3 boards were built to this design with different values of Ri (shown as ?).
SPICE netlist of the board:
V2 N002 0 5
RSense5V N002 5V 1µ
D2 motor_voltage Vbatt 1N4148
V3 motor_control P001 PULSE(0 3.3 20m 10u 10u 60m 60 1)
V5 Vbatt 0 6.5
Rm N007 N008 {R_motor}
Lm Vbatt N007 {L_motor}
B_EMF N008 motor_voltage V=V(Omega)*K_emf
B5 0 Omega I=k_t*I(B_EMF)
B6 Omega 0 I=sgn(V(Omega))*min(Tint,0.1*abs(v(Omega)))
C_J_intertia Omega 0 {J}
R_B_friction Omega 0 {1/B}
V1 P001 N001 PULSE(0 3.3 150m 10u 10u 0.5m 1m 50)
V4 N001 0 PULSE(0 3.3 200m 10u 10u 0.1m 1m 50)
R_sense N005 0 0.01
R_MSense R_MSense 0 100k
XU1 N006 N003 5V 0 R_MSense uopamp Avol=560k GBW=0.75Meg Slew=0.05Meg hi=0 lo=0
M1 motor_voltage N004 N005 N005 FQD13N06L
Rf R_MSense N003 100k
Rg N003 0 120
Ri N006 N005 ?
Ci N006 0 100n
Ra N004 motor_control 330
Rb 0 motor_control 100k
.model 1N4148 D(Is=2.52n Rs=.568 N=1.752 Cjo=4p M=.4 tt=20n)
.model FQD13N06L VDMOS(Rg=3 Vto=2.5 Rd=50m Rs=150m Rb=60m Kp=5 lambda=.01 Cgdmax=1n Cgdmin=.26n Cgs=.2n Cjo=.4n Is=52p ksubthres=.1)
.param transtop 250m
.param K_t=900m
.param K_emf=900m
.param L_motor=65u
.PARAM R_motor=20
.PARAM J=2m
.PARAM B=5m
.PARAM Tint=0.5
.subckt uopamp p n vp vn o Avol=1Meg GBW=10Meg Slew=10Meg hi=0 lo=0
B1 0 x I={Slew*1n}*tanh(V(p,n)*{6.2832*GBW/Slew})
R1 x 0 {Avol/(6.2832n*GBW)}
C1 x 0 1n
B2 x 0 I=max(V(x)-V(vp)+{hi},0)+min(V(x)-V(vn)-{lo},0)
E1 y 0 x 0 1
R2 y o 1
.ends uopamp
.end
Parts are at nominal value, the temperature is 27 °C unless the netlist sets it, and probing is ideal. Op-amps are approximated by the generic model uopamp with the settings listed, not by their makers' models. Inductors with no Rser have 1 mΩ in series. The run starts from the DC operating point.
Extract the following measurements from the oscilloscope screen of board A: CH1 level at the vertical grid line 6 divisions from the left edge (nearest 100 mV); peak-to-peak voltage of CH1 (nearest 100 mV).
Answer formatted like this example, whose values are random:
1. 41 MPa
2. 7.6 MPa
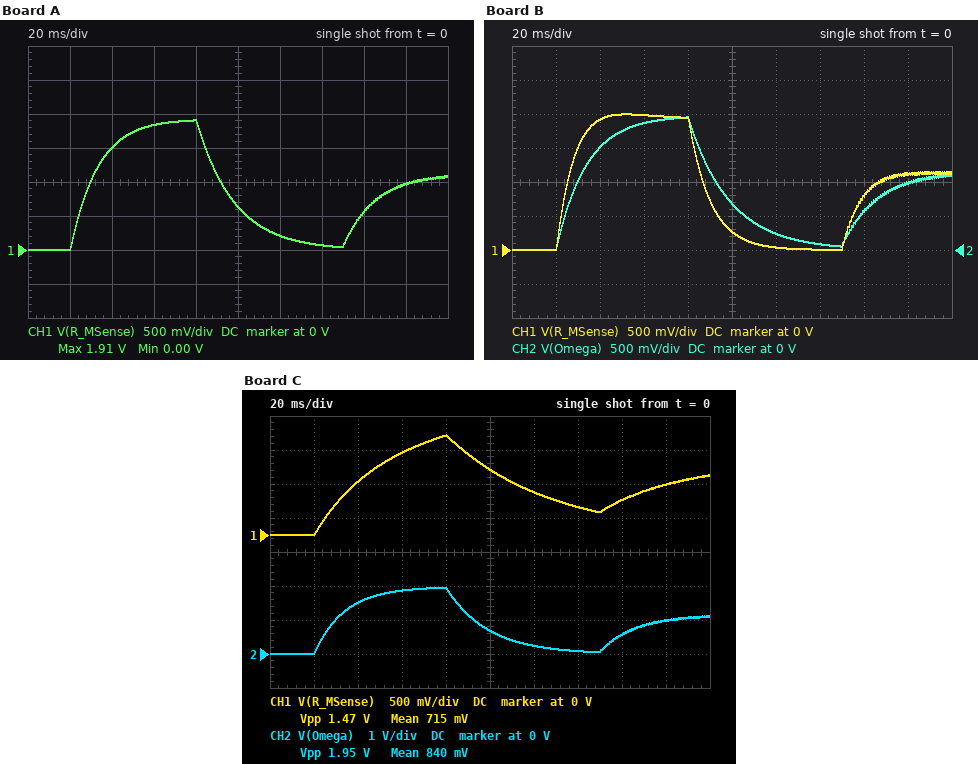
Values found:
1. 200 mV
2. 1.9 V
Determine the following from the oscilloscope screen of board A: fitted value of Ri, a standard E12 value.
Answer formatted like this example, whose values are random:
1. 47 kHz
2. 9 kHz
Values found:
1. 180 kΩ
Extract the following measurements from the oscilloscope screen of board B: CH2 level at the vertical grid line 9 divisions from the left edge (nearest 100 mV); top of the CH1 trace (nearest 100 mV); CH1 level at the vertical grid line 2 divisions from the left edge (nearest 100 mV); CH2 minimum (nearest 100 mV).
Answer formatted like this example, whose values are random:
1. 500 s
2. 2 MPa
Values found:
1. 1.0 V
2. 2.0 V
3. 1.9 V
4. 0 V
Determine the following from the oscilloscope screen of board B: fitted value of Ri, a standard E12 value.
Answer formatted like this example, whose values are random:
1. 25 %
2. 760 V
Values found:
1. 100 kΩ
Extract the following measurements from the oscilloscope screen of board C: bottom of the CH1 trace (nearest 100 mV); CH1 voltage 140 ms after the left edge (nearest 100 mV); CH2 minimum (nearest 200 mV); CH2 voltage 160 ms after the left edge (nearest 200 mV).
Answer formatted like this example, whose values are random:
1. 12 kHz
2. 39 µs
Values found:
1. 0 V
2. 400 mV
3. 0 V
4. 600 mV
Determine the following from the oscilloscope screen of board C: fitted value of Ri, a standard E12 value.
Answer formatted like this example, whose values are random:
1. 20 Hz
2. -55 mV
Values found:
1. 470 kΩ
